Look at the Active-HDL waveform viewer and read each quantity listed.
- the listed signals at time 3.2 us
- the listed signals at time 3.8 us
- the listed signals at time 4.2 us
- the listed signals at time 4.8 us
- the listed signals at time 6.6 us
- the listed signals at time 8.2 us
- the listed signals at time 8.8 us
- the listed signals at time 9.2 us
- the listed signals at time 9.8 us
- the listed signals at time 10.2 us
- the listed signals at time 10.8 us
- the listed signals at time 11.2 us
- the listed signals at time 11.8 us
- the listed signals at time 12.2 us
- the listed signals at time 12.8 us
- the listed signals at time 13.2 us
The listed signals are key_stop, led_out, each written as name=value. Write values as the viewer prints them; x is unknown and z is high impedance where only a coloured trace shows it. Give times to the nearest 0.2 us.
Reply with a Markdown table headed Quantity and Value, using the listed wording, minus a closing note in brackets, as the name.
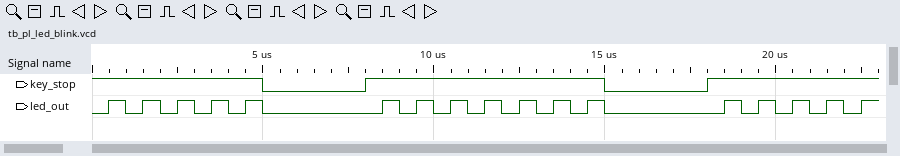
| Quantity | Value |
|---|---|
| the listed signals at time 3.2 us | key_stop=1, led_out=0 |
| the listed signals at time 3.8 us | key_stop=1, led_out=1 |
| the listed signals at time 4.2 us | key_stop=1, led_out=0 |
| the listed signals at time 4.8 us | key_stop=1, led_out=1 |
| the listed signals at time 6.6 us | key_stop=0, led_out=0 |
| the listed signals at time 8.2 us | key_stop=1, led_out=0 |
| the listed signals at time 8.8 us | key_stop=1, led_out=1 |
| the listed signals at time 9.2 us | key_stop=1, led_out=0 |
| the listed signals at time 9.8 us | key_stop=1, led_out=1 |
| the listed signals at time 10.2 us | key_stop=1, led_out=0 |
| the listed signals at time 10.8 us | key_stop=1, led_out=1 |
| the listed signals at time 11.2 us | key_stop=1, led_out=0 |
| the listed signals at time 11.8 us | key_stop=1, led_out=1 |
| the listed signals at time 12.2 us | key_stop=1, led_out=0 |
| the listed signals at time 12.8 us | key_stop=1, led_out=1 |
| the listed signals at time 13.2 us | key_stop=1, led_out=0 |
